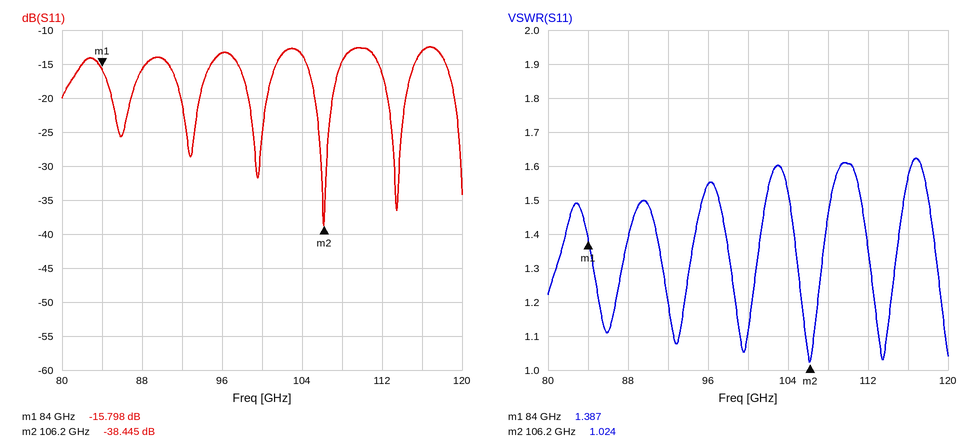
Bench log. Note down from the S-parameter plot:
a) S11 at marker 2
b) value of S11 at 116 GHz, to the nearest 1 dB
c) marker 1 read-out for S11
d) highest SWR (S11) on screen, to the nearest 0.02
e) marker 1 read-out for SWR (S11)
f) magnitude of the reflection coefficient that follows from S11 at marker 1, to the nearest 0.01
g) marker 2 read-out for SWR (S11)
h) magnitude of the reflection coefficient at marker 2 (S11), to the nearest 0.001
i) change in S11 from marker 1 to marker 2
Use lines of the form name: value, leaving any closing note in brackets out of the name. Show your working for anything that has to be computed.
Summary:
S11 at marker 2: -38.445 dB
value of S11 at 116 GHz, to the nearest 1 dB: -13 dB
marker 1 read-out for S11: -15.798 dB
highest SWR (S11) on screen, to the nearest 0.02: 1.62
marker 1 read-out for SWR: 1.387
magnitude of the reflection coefficient that follows from S11 at marker 1, to the nearest 0.01: 10^(-15.798/20) ≈ 0.16
marker 2 read-out for SWR: 1.024
magnitude of the reflection coefficient at marker 2 (S11), to the nearest 0.001: 10^(-38.445/20) ≈ 0.012
change in S11 from marker 1 to marker 2: -38.445 − (-15.798) = -22.647 dB
